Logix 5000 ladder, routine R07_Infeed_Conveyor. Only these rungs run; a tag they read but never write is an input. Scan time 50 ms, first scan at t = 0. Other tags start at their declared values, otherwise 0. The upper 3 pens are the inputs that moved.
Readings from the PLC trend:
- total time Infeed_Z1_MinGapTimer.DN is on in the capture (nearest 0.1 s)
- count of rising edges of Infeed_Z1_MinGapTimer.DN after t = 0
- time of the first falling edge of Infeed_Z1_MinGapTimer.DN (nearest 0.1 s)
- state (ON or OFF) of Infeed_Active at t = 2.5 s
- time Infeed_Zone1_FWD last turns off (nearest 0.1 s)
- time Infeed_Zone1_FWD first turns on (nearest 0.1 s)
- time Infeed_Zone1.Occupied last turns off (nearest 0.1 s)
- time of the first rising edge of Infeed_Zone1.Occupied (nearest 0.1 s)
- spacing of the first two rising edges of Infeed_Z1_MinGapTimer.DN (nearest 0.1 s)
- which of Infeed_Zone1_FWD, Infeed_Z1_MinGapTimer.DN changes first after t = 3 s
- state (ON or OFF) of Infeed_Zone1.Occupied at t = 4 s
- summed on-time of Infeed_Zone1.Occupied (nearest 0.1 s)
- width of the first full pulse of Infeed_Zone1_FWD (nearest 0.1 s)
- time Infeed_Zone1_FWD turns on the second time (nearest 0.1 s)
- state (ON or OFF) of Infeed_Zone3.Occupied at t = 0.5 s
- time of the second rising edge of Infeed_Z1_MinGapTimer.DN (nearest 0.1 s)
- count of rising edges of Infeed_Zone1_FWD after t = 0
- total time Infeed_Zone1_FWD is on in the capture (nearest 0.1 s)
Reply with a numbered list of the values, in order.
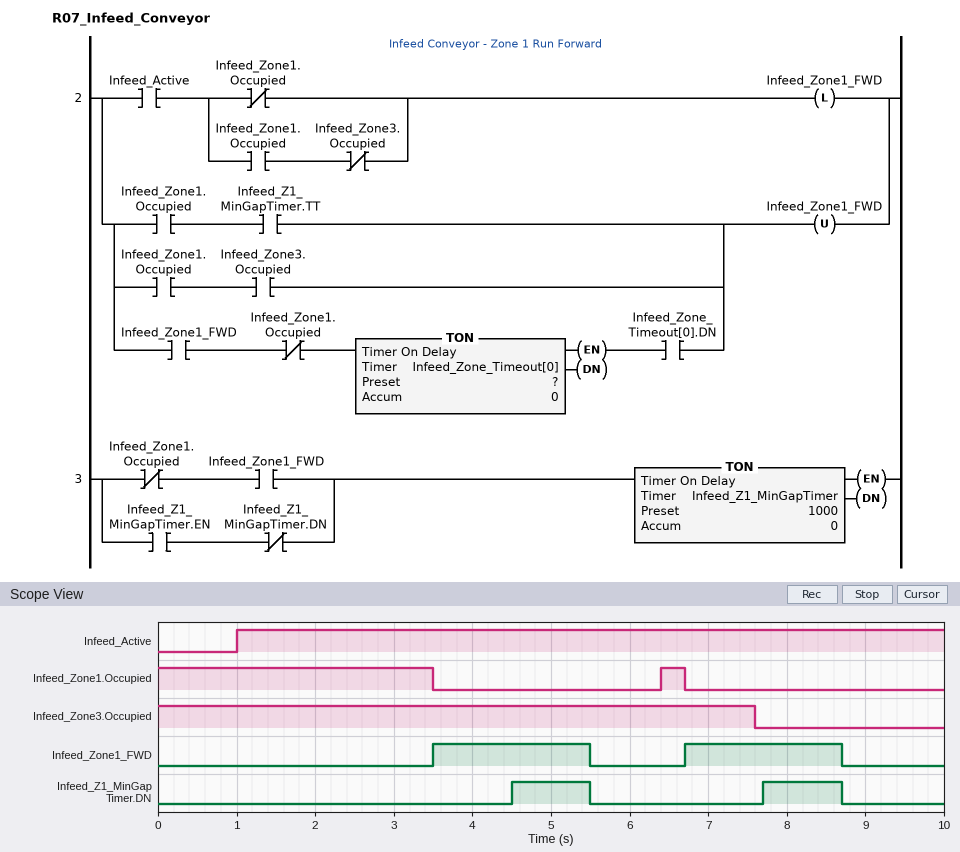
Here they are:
1. 2.0 s
2. 2
3. 5.5 s
4. ON
5. 8.7 s
6. 3.5 s
7. 6.7 s
8. 6.4 s
9. 3.2 s
10. Infeed_Zone1_FWD
11. OFF
12. 3.8 s
13. 2.0 s
14. 6.7 s
15. ON
16. 7.7 s
17. 2
18. 4.0 s
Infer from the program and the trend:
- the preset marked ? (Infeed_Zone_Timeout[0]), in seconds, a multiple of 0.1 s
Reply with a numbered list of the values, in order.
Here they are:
1. 2.0 s
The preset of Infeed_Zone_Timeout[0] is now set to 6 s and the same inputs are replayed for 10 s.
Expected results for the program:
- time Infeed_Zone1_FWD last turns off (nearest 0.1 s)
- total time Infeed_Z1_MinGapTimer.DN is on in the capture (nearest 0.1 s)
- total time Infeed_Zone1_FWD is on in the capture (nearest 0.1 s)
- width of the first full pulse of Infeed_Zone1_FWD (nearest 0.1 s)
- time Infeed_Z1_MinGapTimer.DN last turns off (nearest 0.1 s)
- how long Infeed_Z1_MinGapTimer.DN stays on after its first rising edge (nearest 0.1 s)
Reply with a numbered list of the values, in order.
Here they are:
1. 6.4 s
2. 4.2 s
3. 6.2 s
4. 2.9 s
5. 6.4 s
6. 1.9 s
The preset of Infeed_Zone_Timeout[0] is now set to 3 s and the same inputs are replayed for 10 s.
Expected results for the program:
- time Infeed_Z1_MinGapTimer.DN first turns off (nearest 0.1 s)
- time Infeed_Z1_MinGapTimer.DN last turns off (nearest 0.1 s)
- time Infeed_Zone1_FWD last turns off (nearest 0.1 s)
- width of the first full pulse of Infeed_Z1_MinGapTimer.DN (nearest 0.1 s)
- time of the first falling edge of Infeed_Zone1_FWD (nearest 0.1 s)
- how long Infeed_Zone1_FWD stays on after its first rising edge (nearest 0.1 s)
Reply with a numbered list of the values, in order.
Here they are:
1. 6.4 s
2. 9.7 s
3. 9.7 s
4. 1.9 s
5. 6.4 s
6. 2.9 s
